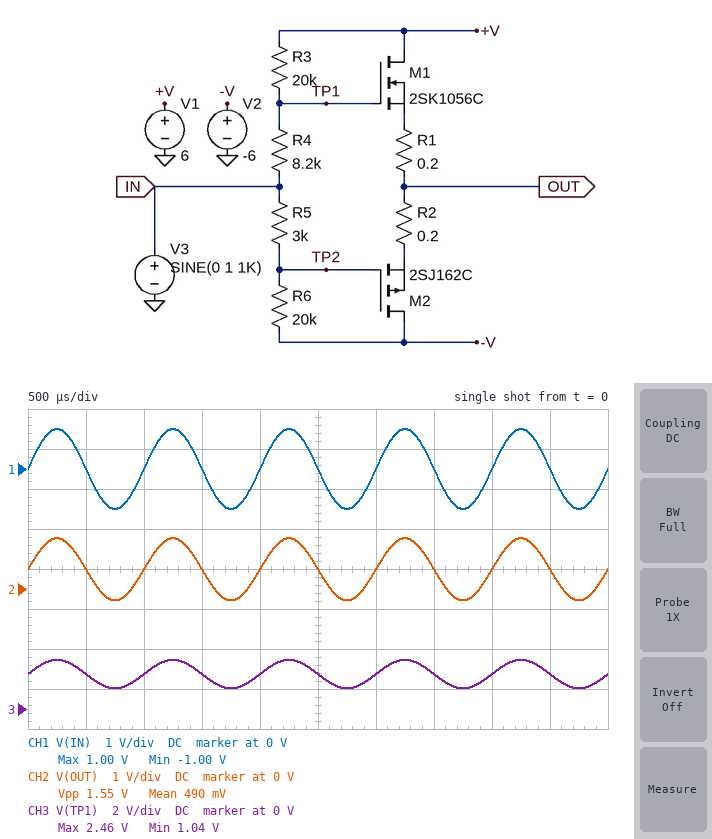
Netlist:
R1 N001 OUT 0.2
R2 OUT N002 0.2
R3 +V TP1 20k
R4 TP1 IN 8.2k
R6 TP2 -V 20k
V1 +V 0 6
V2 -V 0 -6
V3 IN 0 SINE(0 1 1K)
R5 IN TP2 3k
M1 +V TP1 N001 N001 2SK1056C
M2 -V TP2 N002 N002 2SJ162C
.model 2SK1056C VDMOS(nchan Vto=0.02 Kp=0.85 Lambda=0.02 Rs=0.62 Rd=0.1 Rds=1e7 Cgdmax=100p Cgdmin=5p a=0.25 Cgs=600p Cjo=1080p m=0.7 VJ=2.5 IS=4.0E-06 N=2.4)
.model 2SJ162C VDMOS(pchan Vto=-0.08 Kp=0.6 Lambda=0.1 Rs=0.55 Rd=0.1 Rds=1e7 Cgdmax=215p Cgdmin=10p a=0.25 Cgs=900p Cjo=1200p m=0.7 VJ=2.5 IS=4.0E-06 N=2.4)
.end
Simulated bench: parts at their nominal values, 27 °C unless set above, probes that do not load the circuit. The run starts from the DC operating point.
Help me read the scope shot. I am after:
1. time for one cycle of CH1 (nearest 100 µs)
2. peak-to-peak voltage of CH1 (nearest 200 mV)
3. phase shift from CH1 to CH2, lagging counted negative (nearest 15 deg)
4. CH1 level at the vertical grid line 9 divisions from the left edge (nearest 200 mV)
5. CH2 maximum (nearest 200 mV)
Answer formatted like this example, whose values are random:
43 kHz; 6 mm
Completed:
1.0 ms; 2.0 V; 0 deg; 0 V; 1.2 V
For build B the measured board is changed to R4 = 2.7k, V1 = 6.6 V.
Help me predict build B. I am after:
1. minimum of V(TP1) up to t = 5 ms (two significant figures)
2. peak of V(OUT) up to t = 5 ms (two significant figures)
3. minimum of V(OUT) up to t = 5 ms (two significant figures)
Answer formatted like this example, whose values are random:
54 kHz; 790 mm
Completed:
-96 mV; 890 mV; -840 mV
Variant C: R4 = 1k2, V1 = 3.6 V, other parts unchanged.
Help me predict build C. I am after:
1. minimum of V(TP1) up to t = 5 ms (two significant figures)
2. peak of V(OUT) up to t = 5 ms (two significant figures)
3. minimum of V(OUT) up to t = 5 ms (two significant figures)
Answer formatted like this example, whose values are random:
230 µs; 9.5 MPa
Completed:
-740 mV; 630 mV; -1.2 V
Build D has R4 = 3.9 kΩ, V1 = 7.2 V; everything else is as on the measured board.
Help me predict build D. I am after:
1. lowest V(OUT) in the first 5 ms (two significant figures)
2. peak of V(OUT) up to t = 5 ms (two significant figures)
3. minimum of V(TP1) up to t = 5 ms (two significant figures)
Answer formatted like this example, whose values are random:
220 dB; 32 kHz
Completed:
-620 mV; 1.1 V; 340 mV
